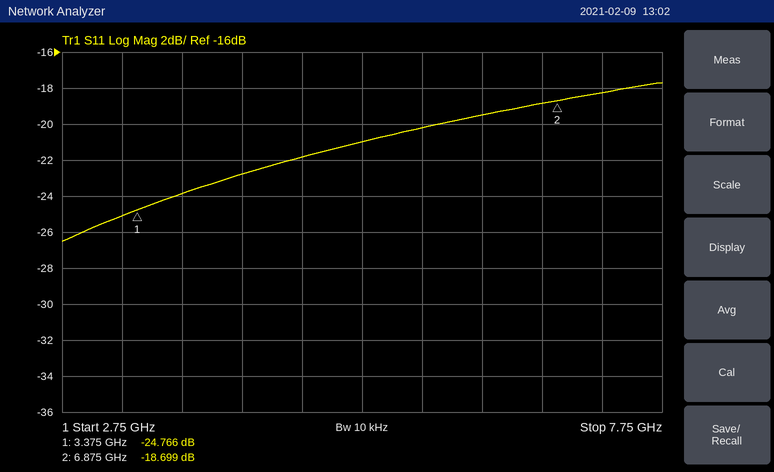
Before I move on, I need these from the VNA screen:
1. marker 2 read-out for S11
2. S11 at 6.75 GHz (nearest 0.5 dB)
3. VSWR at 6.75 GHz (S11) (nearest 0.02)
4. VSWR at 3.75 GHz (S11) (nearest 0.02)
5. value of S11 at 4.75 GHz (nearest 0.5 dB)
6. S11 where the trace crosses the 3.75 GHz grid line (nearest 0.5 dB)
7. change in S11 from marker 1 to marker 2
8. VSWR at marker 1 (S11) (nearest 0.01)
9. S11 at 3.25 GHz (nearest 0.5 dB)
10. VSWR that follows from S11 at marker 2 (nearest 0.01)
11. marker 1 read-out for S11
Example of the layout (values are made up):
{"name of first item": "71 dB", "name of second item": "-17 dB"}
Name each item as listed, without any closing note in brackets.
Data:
{"marker 2 read-out for S11": "-18.699 dB", "S11 at 6.75 GHz": "-19.0 dB", "VSWR at 6.75 GHz (S11)": "1.26", "VSWR at 3.75 GHz (S11)": "1.14", "value of S11 at 4.75 GHz": "-22.0 dB", "S11 where the trace crosses the 3.75 GHz grid line": "-24.0 dB", "change in S11 from marker 1 to marker 2": "6.067 dB", "VSWR at marker 1 (S11)": "1.12", "S11 at 3.25 GHz": "-25.0 dB", "VSWR that follows from S11 at marker 2": "1.26", "marker 1 read-out for S11": "-24.766 dB"}
